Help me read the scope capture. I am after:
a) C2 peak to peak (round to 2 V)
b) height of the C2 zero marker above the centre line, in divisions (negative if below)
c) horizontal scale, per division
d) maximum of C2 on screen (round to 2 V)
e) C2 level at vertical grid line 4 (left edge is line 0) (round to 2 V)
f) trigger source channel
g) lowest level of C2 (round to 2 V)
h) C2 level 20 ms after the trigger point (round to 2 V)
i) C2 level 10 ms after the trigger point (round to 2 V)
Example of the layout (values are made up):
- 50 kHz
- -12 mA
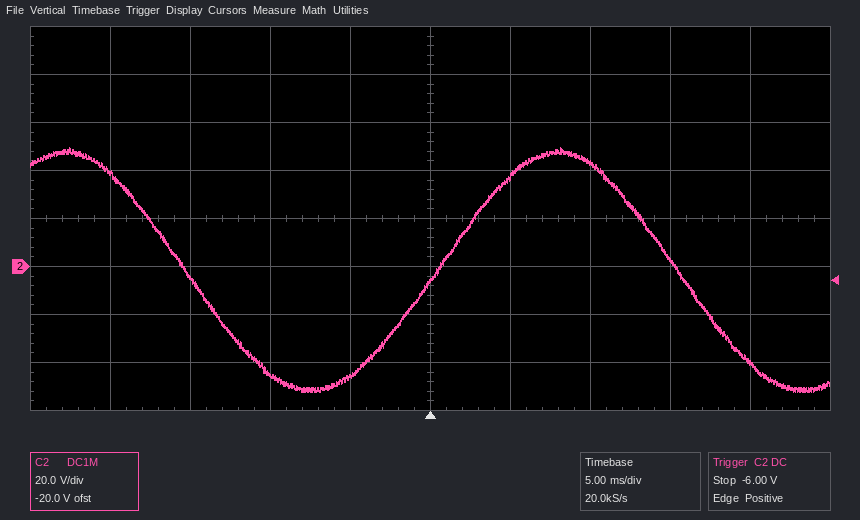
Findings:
- 102 V
- -1.0 div
- 5 ms
- 50 V
- -46 V
- C2
- -52 V
- -40 V
- 44 V
